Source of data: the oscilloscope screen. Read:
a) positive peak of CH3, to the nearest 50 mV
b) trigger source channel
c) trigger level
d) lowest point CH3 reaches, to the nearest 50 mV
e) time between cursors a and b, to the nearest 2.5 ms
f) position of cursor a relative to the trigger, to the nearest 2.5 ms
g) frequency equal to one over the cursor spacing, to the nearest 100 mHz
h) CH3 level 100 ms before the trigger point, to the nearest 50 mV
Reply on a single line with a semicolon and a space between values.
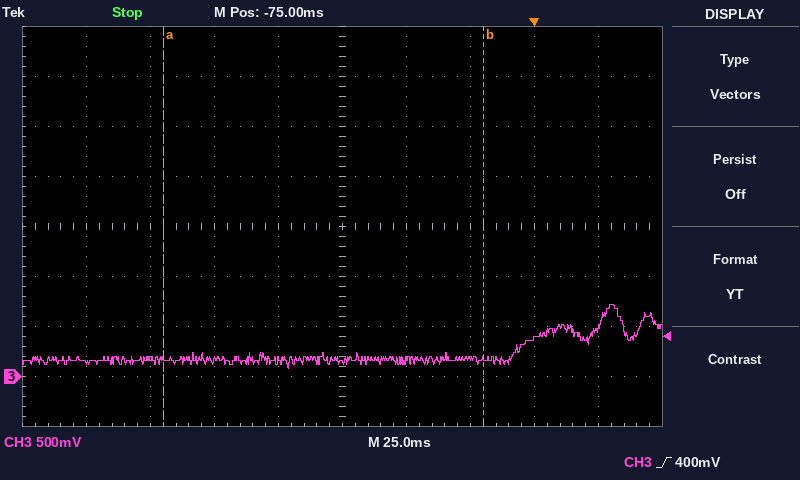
700 mV; CH3; 400 mV; 100 mV; 125.0 ms; -145.0 ms; 8.0 Hz; 150 mV
